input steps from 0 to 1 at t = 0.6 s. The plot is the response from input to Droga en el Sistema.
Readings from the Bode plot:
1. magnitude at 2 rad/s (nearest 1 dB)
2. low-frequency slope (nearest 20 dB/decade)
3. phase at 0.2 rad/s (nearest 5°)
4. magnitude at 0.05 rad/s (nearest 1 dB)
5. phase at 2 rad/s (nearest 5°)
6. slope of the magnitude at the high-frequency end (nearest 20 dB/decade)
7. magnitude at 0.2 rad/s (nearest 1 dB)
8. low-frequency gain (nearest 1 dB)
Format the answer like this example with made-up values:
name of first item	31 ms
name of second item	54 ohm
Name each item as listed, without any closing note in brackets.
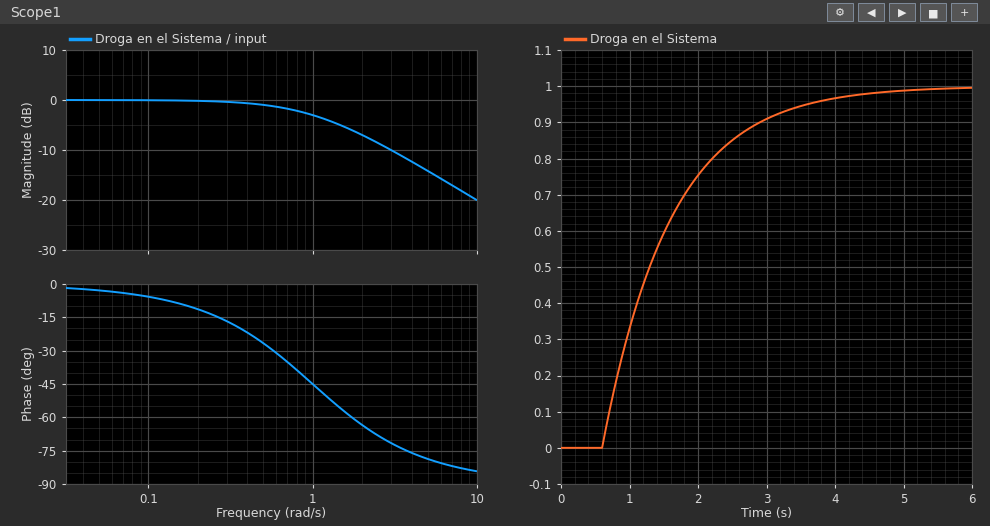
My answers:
magnitude at 2 rad/s	-7 dB
low-frequency slope	0 dB/decade
phase at 0.2 rad/s	-10°
magnitude at 0.05 rad/s	0 dB
phase at 2 rad/s	-65°
slope of the magnitude at the high-frequency end	-20 dB/decade
magnitude at 0.2 rad/s	0 dB
low-frequency gain	0 dB
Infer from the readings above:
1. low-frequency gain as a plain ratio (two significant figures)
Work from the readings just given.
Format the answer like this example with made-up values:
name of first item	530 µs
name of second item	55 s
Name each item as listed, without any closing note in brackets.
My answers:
low-frequency gain as a plain ratio	1.0
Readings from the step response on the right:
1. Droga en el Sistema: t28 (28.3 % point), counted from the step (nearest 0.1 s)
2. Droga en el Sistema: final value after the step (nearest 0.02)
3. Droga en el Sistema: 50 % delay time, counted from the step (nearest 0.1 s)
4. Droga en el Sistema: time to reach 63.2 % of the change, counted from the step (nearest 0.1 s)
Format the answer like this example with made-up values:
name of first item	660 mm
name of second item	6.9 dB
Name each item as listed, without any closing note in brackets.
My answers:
Droga en el Sistema: t28 (28.3 % point), counted from the step	0.3 s
Droga en el Sistema: final value after the step	1.00
Droga en el Sistema: 50 % delay time, counted from the step	0.7 s
Droga en el Sistema: time to reach 63.2 % of the change, counted from the step	1.0 s
